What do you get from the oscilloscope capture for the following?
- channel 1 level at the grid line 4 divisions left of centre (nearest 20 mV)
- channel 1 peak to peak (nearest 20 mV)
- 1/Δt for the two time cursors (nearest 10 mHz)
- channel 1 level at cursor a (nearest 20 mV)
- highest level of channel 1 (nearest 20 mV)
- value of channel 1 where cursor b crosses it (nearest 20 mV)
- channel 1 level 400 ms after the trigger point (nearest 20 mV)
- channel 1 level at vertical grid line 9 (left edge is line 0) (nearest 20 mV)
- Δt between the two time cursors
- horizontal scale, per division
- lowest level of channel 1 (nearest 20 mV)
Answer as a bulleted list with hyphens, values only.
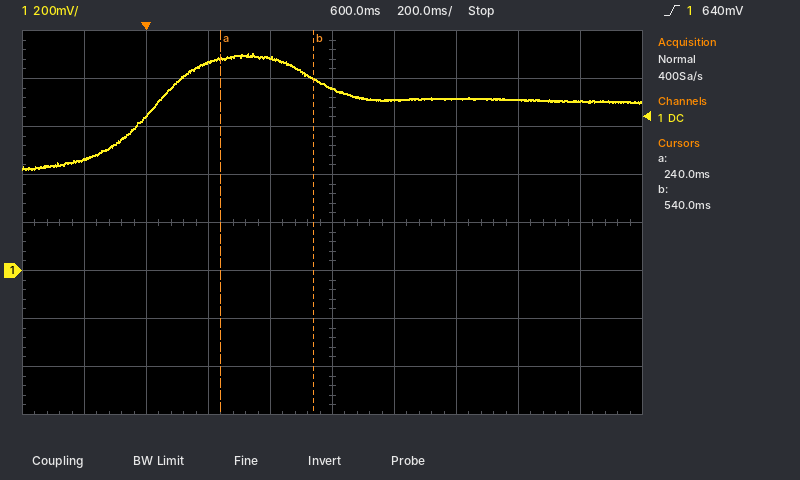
- 460 mV
- 480 mV
- 3.33 Hz
- 880 mV
- 900 mV
- 800 mV
- 880 mV
- 700 mV
- 300 ms
- 200 ms
- 420 mV
